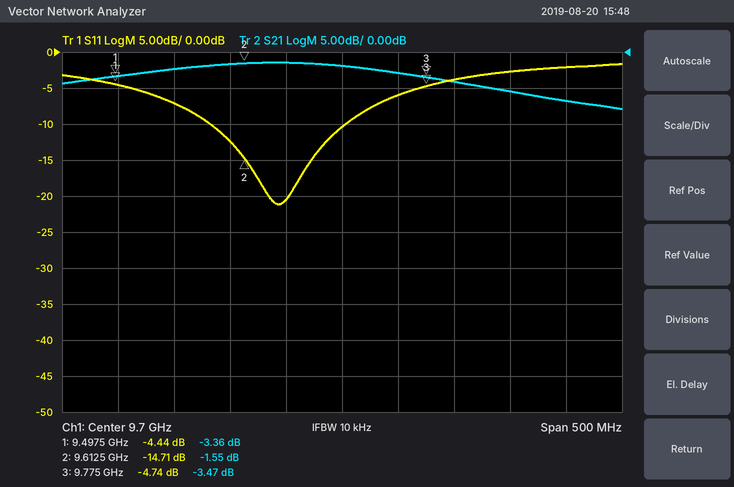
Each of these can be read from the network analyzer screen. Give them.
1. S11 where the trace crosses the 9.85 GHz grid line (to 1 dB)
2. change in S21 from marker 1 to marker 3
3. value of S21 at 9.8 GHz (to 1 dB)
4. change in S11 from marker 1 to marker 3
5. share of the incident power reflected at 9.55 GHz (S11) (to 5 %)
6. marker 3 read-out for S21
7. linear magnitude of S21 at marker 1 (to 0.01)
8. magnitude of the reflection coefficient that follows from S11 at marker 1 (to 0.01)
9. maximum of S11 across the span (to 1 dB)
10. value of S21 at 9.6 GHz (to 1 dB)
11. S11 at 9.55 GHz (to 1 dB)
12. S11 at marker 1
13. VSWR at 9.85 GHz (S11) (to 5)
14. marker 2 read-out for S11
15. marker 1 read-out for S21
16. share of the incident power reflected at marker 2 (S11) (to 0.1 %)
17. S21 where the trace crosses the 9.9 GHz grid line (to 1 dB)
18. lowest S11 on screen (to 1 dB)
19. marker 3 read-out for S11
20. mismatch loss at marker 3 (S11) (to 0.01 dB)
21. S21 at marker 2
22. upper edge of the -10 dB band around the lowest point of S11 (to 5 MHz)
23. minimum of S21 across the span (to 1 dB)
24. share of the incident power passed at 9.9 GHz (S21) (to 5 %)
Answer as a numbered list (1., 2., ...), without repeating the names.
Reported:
1. -3 dB
2. -0.11 dB
3. -4 dB
4. -0.30 dB
5. 20 %
6. -3.47 dB
7. 0.68
8. 0.60
9. -2 dB
10. -2 dB
11. -7 dB
12. -4.44 dB
13. 5
14. -14.71 dB
15. -3.36 dB
16. 3.4 %
17. -7 dB
18. -21 dB
19. -4.74 dB
20. 1.78 dB
21. -1.55 dB
22. 9.705 GHz
23. -8 dB
24. 20 %
